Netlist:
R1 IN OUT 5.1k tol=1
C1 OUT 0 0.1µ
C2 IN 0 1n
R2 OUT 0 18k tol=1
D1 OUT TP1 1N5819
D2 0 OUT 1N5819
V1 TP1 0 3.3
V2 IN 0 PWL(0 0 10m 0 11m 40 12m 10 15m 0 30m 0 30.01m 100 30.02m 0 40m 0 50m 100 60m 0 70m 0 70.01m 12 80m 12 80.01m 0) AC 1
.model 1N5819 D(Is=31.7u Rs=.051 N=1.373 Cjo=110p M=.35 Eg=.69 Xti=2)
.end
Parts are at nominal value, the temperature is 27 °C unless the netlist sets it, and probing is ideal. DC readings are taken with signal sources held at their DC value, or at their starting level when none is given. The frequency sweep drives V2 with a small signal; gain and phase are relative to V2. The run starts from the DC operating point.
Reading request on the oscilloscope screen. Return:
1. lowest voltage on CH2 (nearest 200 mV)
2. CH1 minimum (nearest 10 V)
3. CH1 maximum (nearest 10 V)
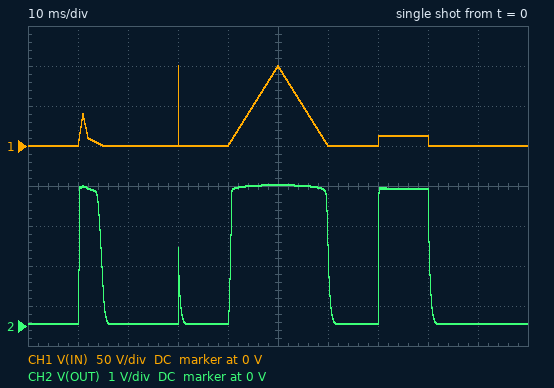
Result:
0 V
0 V
100 V
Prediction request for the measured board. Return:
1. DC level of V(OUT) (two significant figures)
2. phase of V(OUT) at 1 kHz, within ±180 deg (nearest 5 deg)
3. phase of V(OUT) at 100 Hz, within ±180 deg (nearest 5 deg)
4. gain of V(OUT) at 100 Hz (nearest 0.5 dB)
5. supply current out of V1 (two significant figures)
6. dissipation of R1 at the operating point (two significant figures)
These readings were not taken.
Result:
40 mV
-50 deg
-5 deg
-9.0 dB
32 µA
320 nW
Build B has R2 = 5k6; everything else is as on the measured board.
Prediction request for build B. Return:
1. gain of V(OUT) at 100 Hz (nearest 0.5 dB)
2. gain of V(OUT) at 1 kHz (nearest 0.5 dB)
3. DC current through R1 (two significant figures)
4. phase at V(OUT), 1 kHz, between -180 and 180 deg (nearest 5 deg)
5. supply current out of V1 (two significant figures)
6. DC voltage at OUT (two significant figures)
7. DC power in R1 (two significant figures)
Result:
-11.5 dB
-14.0 dB
6.5 µA
-40 deg
32 µA
33 mV
220 nW
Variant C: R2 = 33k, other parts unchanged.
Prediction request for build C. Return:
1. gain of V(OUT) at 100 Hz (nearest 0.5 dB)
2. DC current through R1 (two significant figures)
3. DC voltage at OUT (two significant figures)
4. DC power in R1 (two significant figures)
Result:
-8.0 dB
8.3 µA
42 mV
350 nW
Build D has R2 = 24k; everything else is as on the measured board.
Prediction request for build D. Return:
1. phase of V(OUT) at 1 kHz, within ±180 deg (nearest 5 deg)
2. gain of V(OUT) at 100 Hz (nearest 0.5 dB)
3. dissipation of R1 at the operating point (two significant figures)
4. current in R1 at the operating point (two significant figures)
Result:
-50 deg
-8.5 dB
340 nW
8.1 µA
